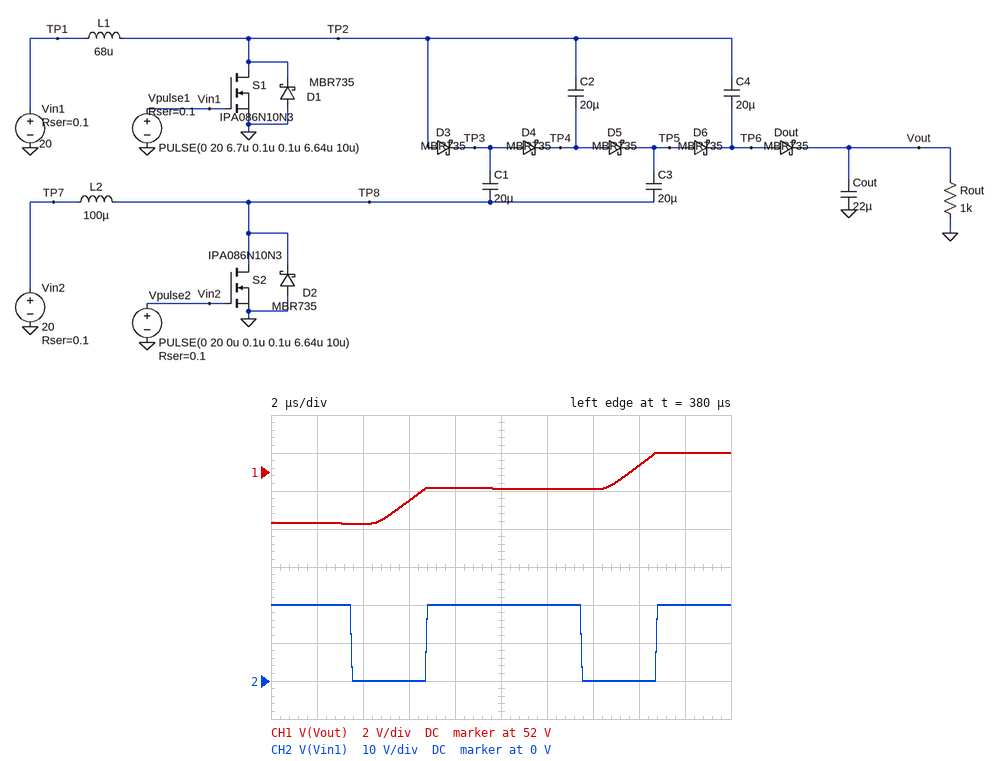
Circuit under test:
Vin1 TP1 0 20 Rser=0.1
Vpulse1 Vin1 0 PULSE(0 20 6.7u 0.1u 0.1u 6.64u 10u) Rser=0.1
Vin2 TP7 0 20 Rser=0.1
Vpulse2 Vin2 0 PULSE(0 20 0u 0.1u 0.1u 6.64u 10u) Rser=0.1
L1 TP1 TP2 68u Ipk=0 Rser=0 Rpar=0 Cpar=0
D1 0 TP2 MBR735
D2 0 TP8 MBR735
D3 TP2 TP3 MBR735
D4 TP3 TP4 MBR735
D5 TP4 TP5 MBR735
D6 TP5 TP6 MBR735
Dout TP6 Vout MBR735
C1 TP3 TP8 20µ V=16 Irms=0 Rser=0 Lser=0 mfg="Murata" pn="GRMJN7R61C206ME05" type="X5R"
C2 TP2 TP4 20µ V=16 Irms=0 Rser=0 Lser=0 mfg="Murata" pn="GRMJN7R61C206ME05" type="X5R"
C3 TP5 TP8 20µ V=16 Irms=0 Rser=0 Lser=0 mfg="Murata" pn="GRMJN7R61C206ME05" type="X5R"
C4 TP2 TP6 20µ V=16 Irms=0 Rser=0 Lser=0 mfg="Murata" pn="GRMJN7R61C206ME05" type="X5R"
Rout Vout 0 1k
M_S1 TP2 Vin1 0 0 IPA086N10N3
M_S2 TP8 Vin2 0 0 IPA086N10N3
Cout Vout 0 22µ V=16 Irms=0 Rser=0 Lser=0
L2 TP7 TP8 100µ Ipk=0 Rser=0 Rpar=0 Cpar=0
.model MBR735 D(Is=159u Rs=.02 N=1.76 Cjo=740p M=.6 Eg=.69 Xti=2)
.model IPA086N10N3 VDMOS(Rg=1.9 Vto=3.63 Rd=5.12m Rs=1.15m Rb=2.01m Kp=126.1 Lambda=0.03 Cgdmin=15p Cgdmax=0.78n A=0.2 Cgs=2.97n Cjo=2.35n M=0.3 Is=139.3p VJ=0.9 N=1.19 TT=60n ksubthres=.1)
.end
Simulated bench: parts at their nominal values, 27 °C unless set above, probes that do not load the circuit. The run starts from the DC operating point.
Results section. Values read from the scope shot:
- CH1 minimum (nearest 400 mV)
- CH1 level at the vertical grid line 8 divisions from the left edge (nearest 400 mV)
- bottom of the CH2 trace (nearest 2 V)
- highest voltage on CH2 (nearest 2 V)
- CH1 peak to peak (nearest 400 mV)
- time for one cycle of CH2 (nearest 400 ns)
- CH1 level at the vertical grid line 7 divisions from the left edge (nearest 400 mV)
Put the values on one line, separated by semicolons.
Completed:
49.2 V; 52.4 V; 0 V; 20 V; 3.6 V; 10.0 µs; 51.2 V
